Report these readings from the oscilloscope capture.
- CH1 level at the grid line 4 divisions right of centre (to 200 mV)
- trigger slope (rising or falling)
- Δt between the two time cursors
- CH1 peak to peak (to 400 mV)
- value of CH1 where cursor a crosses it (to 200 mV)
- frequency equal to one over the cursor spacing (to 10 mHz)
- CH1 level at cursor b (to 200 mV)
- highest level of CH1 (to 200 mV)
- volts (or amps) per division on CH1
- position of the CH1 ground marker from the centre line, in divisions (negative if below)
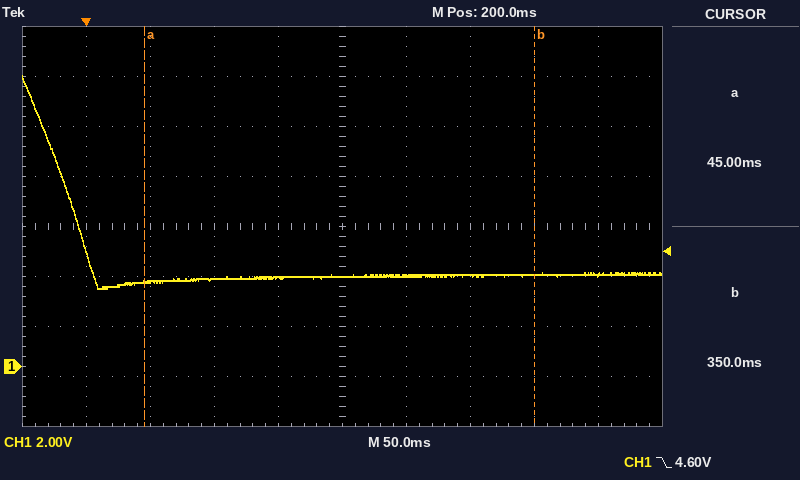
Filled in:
3.6 V
falling
305 ms
8.4 V
3.4 V
3.28 Hz
3.6 V
11.6 V
2 V
-2.8 div
